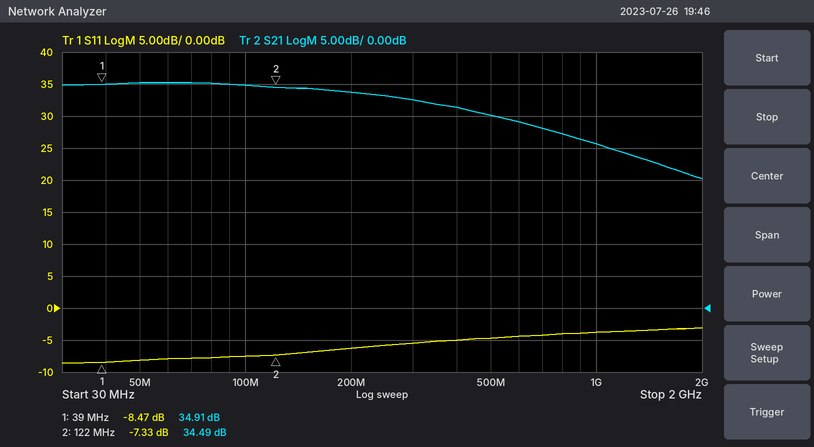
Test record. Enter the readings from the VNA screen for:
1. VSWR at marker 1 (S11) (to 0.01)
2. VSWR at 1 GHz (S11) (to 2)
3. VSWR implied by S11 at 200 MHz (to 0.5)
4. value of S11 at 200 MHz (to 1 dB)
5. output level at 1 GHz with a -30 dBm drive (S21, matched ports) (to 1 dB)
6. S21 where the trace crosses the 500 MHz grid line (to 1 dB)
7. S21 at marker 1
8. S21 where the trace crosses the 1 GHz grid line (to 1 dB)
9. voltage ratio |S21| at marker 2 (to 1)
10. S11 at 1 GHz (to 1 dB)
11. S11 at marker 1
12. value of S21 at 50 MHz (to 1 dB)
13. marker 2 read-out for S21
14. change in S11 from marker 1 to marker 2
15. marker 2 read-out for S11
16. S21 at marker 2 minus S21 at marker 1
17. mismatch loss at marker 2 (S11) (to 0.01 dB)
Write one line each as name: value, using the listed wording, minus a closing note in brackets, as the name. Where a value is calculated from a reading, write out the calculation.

VSWR at marker 1 (S11): (1 + 0.3771)/(1 − 0.3771) ≈ 2.21
VSWR at 1 GHz (S11): |Γ| = 10^(-4/20) = 0.6310; VSWR = (1 + 0.6310)/(1 − 0.6310) ≈ 4
VSWR implied by S11 at 200 MHz: |Γ| = 10^(-6/20) = 0.5012; VSWR = (1 + 0.5012)/(1 − 0.5012) ≈ 3.0
value of S11 at 200 MHz: -6 dB
output level at 1 GHz with a -30 dBm drive (S21, matched ports): -30 dBm + (26 dB) = -4 dBm
S21 where the trace crosses the 500 MHz grid line: 30 dB
S21 at marker 1: 34.91 dB
S21 where the trace crosses the 1 GHz grid line: 26 dB
voltage ratio |S21| at marker 2: 10^(34.49/20) ≈ 53
S11 at 1 GHz: -4 dB
S11 at marker 1: -8.47 dB
value of S21 at 50 MHz: 35 dB
marker 2 read-out for S21: 34.49 dB
change in S11 from marker 1 to marker 2: -7.33 − (-8.47) = 1.14 dB
marker 2 read-out for S11: -7.33 dB
S21 at marker 2 minus S21 at marker 1: 34.49 − (34.91) = -0.42 dB
mismatch loss at marker 2 (S11): −10 log10(1 − 10^(-7.33/10)) ≈ 0.89 dB
